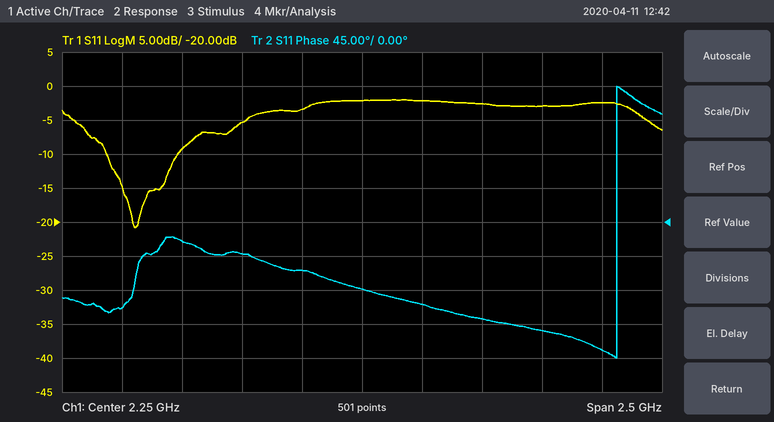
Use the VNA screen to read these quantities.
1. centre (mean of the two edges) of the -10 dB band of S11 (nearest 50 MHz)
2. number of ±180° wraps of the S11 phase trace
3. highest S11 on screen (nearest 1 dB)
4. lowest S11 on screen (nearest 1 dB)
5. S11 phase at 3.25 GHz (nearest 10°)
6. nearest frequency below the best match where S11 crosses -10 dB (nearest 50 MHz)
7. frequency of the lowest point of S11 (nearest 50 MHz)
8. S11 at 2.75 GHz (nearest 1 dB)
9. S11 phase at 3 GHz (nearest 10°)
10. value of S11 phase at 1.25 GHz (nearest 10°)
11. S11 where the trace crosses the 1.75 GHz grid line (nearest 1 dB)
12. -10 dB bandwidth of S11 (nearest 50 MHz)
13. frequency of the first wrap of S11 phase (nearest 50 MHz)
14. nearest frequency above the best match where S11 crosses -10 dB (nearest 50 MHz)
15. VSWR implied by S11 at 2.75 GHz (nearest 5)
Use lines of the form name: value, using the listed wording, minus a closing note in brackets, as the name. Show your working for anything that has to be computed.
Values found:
centre (mean of the two edges) of the -10 dB band of S11: 1.35 GHz
number of ±180° wraps of the S11 phase trace: 1
highest S11 on screen: -2 dB
lowest S11 on screen: -21 dB
S11 phase at 3.25 GHz: -170°
nearest frequency below the best match where S11 crosses -10 dB: 1.20 GHz
frequency of the lowest point of S11: 1.30 GHz
S11 at 2.75 GHz: -3 dB
S11 phase at 3 GHz: -140°
value of S11 phase at 1.25 GHz: -110°
S11 where the trace crosses the 1.75 GHz grid line: -5 dB
-10 dB bandwidth of S11: 1.50 GHz − 1.20 GHz = 300 MHz
frequency of the first wrap of S11 phase: 3.30 GHz
nearest frequency above the best match where S11 crosses -10 dB: 1.50 GHz
VSWR implied by S11 at 2.75 GHz: |Γ| = 10^(-3/20) = 0.7079; VSWR = (1 + 0.7079)/(1 − 0.7079) ≈ 5.85, so 5 to the nearest 5
